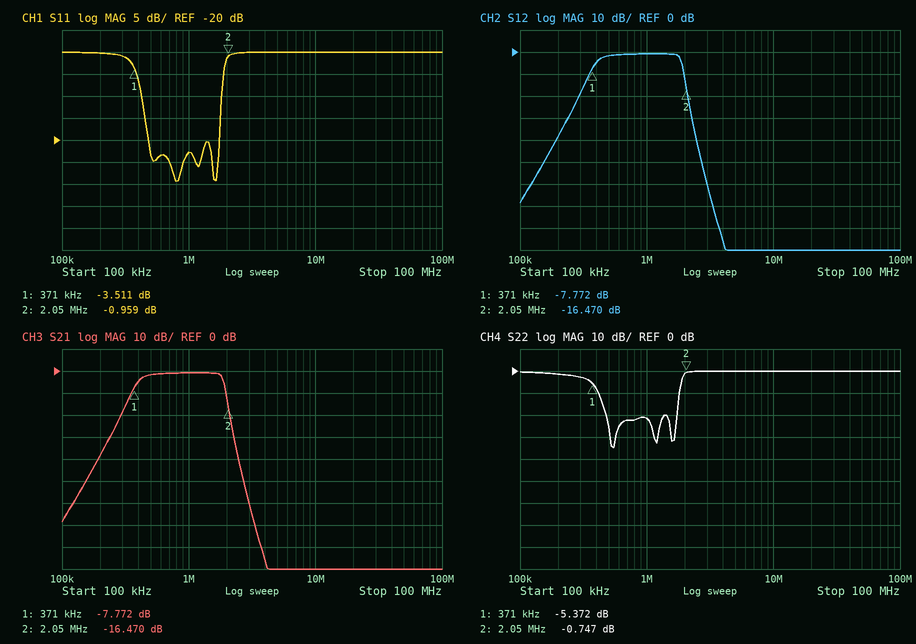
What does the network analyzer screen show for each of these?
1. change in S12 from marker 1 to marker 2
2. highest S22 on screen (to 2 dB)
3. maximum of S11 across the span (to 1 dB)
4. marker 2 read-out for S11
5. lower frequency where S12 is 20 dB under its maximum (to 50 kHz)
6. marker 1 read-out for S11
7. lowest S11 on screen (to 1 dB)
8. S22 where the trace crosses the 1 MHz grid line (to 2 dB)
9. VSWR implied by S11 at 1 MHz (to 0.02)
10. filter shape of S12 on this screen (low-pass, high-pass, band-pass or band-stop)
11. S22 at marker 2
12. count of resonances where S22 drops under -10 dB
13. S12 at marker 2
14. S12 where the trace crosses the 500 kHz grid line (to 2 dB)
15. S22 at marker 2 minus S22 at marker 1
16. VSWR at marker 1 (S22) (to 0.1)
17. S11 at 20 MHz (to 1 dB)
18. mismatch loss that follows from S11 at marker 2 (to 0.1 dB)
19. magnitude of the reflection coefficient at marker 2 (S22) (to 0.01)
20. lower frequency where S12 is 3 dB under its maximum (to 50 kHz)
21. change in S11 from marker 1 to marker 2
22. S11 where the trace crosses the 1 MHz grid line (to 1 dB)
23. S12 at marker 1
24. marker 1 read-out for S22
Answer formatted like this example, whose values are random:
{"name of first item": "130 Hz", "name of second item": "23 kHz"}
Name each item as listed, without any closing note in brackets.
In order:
{"change in S12 from marker 1 to marker 2": "-8.698 dB", "highest S22 on screen": "0 dB", "maximum of S11 across the span": "0 dB", "marker 2 read-out for S11": "-0.959 dB", "lower frequency where S12 is 20 dB under its maximum": "300 kHz", "marker 1 read-out for S11": "-3.511 dB", "lowest S11 on screen": "-29 dB", "S22 where the trace crosses the 1 MHz grid line": "-22 dB", "VSWR implied by S11 at 1 MHz": "1.16", "filter shape of S12 on this screen": "band-pass", "S22 at marker 2": "-0.747 dB", "count of resonances where S22 drops under -10 dB": "3", "S12 at marker 2": "-16.470 dB", "S12 where the trace crosses the 500 kHz grid line": "-2 dB", "S22 at marker 2 minus S22 at marker 1": "4.625 dB", "VSWR at marker 1 (S22)": "3.3", "S11 at 20 MHz": "0 dB", "mismatch loss that follows from S11 at marker 2": "7.0 dB", "magnitude of the reflection coefficient at marker 2 (S22)": "0.92", "lower frequency where S12 is 3 dB under its maximum": "400 kHz", "change in S11 from marker 1 to marker 2": "2.552 dB", "S11 where the trace crosses the 1 MHz grid line": "-23 dB", "S12 at marker 1": "-7.772 dB", "marker 1 read-out for S22": "-5.372 dB"}
